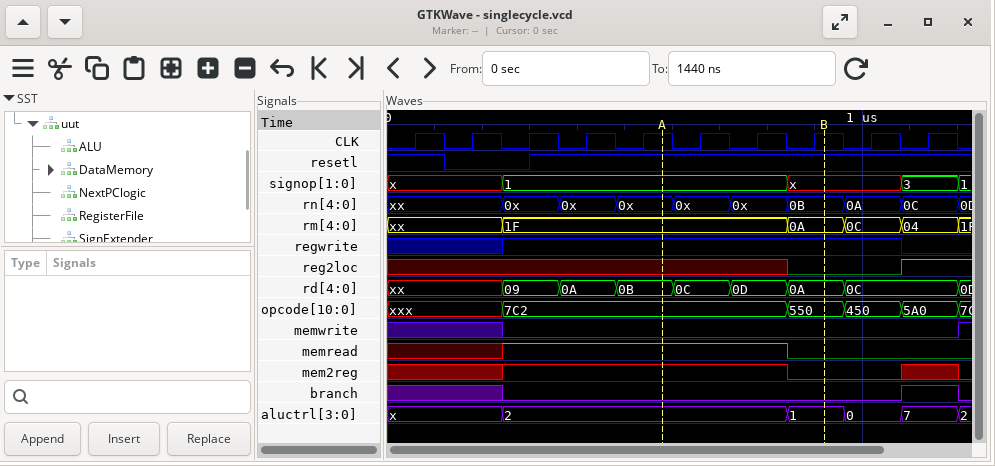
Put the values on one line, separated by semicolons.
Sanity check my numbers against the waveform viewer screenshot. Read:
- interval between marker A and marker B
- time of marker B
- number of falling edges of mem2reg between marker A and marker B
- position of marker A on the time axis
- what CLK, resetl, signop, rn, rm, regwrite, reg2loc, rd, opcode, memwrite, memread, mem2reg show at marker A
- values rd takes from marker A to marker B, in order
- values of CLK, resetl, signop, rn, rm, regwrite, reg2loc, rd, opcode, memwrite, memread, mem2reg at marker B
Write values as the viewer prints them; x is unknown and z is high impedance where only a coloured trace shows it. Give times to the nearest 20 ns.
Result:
340 ns; 920 ns; 1; 580 ns; CLK=1, resetl=1, signop=1, rn=0x, rm=1F, regwrite=1, reg2loc=x, rd=0B, opcode=7C2, memwrite=0, memread=1, mem2reg=1; 0B, 0C, 0D, 0A; CLK=1, resetl=1, signop=x, rn=0B, rm=0A, regwrite=1, reg2loc=0, rd=0A, opcode=550, memwrite=0, memread=0, mem2reg=0
